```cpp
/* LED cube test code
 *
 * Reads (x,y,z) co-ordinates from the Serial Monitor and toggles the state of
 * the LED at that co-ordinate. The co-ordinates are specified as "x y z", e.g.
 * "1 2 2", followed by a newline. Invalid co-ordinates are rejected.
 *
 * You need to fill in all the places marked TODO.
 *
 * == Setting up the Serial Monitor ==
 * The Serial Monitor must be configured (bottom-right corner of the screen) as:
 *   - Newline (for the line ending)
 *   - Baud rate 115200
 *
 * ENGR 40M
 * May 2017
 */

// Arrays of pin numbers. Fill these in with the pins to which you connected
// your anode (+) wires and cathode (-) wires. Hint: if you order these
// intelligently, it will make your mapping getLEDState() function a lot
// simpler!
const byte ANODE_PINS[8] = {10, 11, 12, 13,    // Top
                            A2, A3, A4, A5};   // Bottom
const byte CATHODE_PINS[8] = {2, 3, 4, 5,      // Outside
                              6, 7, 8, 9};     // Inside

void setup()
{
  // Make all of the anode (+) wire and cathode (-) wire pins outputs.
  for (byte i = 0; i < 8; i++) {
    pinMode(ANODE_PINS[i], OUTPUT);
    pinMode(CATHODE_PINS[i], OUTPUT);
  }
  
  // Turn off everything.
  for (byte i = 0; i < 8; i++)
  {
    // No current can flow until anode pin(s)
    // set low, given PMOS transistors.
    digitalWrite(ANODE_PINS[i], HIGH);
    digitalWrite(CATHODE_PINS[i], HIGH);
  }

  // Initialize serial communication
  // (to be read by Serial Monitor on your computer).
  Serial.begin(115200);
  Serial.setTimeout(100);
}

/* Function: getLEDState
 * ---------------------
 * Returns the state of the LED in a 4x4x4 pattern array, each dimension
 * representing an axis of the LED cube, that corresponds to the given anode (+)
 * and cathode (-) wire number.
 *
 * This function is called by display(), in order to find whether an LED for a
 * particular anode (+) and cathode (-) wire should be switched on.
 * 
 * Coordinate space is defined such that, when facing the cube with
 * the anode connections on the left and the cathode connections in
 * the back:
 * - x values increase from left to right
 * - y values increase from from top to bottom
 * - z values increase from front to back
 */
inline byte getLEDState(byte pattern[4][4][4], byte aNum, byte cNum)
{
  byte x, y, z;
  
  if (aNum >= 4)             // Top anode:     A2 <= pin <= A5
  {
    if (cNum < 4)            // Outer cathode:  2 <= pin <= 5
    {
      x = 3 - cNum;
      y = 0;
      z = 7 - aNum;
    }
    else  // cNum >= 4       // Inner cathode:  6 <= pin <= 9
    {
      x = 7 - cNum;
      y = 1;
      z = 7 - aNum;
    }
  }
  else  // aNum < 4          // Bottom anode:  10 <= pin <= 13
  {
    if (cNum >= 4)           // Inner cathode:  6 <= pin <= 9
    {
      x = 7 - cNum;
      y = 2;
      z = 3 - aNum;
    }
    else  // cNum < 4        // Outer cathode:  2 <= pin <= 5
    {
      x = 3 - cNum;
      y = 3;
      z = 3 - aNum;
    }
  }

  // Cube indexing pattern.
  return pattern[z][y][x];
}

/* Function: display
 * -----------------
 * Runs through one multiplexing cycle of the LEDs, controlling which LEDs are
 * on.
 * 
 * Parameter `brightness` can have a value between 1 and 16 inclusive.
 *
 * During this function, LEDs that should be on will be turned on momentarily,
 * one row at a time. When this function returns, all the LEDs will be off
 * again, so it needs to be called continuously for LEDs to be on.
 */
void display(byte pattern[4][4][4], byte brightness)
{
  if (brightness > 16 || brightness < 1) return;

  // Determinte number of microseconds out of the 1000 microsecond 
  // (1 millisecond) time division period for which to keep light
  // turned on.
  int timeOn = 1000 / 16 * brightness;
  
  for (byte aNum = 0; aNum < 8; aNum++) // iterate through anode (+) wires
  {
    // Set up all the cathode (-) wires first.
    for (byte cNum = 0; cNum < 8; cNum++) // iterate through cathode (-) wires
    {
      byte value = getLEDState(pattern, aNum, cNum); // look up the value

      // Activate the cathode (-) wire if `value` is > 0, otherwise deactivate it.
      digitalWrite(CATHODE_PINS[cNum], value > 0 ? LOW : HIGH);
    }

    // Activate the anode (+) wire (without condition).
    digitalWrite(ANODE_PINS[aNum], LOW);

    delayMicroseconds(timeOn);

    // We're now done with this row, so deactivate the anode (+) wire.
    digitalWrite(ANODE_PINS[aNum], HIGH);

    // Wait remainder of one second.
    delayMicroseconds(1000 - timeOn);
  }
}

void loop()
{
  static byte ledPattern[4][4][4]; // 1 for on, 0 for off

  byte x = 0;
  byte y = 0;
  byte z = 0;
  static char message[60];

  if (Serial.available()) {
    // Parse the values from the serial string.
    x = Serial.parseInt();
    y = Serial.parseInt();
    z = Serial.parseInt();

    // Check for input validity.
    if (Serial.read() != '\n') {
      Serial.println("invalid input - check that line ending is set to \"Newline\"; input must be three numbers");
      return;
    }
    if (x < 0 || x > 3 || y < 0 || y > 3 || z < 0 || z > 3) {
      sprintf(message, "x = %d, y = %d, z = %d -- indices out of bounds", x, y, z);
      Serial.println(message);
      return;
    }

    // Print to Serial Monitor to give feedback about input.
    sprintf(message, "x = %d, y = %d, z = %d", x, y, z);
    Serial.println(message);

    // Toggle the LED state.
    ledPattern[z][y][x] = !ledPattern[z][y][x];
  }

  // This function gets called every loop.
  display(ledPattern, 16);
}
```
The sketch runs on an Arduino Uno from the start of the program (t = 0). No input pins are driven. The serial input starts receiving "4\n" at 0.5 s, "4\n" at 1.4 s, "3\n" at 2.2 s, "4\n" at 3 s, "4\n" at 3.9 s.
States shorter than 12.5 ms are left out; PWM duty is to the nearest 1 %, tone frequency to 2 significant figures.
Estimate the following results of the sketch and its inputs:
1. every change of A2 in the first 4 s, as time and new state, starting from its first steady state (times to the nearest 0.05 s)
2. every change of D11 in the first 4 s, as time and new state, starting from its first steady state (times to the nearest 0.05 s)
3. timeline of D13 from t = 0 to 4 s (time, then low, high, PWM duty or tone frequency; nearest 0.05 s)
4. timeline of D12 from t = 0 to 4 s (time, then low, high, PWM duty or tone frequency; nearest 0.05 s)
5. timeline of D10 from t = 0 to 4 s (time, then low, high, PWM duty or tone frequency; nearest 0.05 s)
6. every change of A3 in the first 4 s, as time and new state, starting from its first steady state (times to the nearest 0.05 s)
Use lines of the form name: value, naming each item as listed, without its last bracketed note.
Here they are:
every change of A2 in the first 4 s, as time and new state, starting from its first steady state: 0 s tone 120 Hz; 0.5 s high; 0.7 s tone 120 Hz; 1.4 s high; 1.6 s tone 120 Hz; 2.2 s high; 2.4 s tone 120 Hz; 3 s high; 3.2 s tone 120 Hz; 3.9 s high
every change of D11 in the first 4 s, as time and new state, starting from its first steady state: 0 s tone 120 Hz; 0.5 s high; 0.7 s tone 120 Hz; 1.4 s high; 1.6 s tone 120 Hz; 2.2 s high; 2.4 s tone 120 Hz; 3 s high; 3.2 s tone 120 Hz; 3.9 s high
timeline of D13 from t = 0 to 4 s: 0 s tone 120 Hz; 0.5 s high; 0.7 s tone 120 Hz; 1.4 s high; 1.6 s tone 120 Hz; 2.2 s high; 2.4 s tone 120 Hz; 3 s high; 3.2 s tone 120 Hz; 3.9 s high
timeline of D12 from t = 0 to 4 s: 0 s tone 120 Hz; 0.5 s high; 0.7 s tone 120 Hz; 1.4 s high; 1.6 s tone 120 Hz; 2.2 s high; 2.4 s tone 120 Hz; 3 s high; 3.2 s tone 120 Hz; 3.9 s high
timeline of D10 from t = 0 to 4 s: 0 s tone 120 Hz; 0.5 s high; 0.7 s tone 120 Hz; 1.4 s high; 1.6 s tone 120 Hz; 2.2 s high; 2.4 s tone 120 Hz; 3 s high; 3.2 s tone 120 Hz; 3.9 s high
every change of A3 in the first 4 s, as time and new state, starting from its first steady state: 0 s tone 120 Hz; 0.5 s high; 0.7 s tone 120 Hz; 1.4 s high; 1.6 s tone 120 Hz; 2.2 s high; 2.4 s tone 120 Hz; 3 s high; 3.2 s tone 120 Hz; 3.9 s high
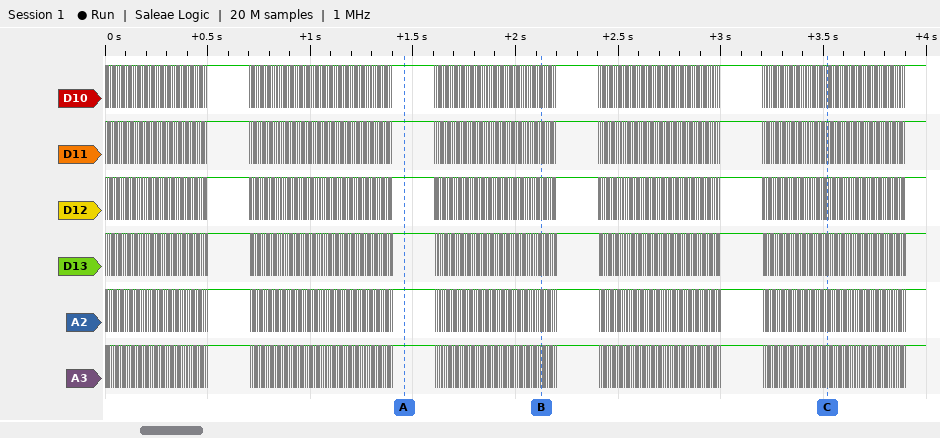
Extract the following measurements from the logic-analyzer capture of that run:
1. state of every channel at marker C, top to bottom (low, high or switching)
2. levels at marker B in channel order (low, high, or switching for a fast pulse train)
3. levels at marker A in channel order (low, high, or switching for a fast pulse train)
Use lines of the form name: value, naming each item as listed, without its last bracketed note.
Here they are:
state of every channel at marker C, top to bottom: D10 switching, D11 switching, D12 switching, D13 switching, A2 switching, A3 switching
levels at marker B in channel order: D10 switching, D11 switching, D12 switching, D13 switching, A2 switching, A3 switching
levels at marker A in channel order: D10 high, D11 high, D12 high, D13 high, A2 high, A3 high
